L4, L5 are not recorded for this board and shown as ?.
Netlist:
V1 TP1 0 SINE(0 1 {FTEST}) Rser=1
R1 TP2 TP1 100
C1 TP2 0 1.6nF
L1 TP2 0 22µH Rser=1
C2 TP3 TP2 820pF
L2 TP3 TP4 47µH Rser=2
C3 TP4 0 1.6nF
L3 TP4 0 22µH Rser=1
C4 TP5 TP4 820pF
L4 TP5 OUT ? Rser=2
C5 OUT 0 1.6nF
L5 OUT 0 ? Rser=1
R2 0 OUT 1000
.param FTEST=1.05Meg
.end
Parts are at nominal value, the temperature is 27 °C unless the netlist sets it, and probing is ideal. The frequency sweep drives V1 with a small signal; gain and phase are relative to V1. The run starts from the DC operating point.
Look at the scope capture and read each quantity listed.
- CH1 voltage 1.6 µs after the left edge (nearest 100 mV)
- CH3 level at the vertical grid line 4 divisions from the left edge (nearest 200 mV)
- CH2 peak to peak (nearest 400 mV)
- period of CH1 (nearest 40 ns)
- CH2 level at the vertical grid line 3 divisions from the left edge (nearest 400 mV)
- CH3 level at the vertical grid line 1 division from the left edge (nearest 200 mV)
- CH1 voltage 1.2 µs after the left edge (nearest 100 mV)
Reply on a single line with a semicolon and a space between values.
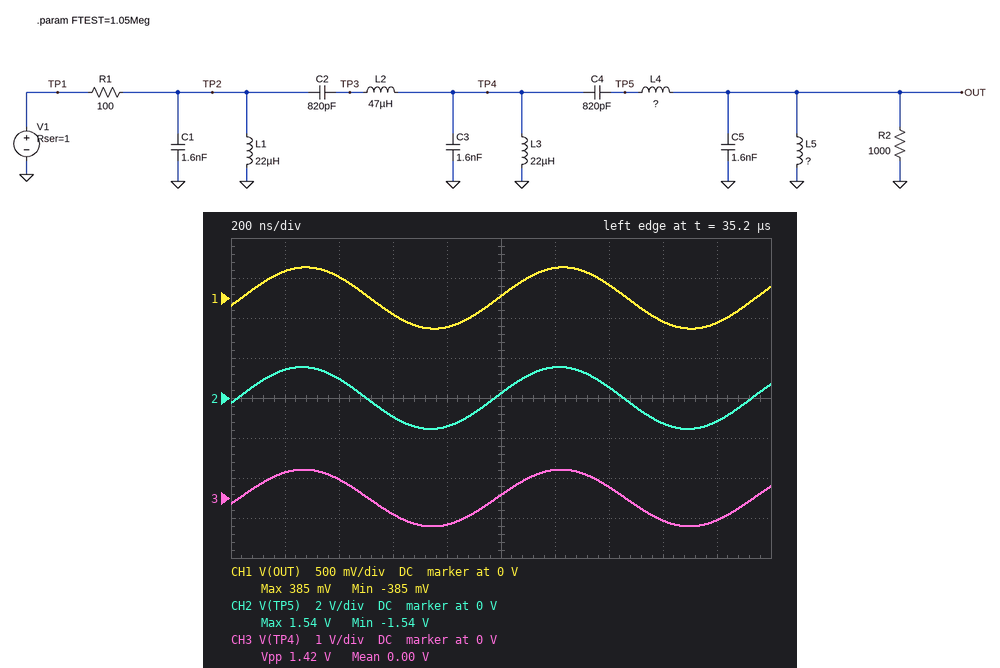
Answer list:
-300 mV; -600 mV; 3.2 V; 960 ns; -800 mV; 600 mV; 400 mV
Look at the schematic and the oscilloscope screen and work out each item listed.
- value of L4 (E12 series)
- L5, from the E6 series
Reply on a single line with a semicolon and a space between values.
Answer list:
39 µH; 6.8 µH
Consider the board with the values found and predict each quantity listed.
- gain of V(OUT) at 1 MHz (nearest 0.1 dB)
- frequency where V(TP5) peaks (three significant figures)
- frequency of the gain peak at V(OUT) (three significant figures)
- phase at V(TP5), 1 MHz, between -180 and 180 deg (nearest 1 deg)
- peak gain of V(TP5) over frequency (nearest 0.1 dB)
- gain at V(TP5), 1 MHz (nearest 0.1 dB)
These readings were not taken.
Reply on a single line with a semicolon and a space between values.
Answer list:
-8.5 dB; 1.30 MHz; 1.31 MHz; 4 deg; 8.5 dB; 4.1 dB
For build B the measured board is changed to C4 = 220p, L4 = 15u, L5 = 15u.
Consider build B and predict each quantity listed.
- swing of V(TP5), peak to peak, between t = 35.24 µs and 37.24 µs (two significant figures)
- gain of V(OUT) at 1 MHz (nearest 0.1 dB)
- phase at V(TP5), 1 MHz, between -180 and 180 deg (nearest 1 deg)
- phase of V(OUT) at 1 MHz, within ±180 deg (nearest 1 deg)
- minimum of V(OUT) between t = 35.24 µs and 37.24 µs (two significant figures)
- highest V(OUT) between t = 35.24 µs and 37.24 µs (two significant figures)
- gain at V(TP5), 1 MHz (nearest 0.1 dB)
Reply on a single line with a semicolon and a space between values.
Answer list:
1.6 V; 0.3 dB; 12 deg; 6 deg; -830 mV; 830 mV; 0.8 dB
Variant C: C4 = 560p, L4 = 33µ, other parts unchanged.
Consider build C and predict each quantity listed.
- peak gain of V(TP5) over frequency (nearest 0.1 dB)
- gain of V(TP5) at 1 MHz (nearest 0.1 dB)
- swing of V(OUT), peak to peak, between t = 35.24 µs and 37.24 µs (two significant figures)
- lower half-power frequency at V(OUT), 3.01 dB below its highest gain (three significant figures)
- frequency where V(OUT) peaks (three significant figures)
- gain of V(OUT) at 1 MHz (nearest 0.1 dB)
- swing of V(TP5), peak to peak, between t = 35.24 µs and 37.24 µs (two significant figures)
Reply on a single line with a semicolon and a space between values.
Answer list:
8.9 dB; 6.4 dB; 1.1 V; 1.27 MHz; 1.33 MHz; -5.1 dB; 3.8 V
